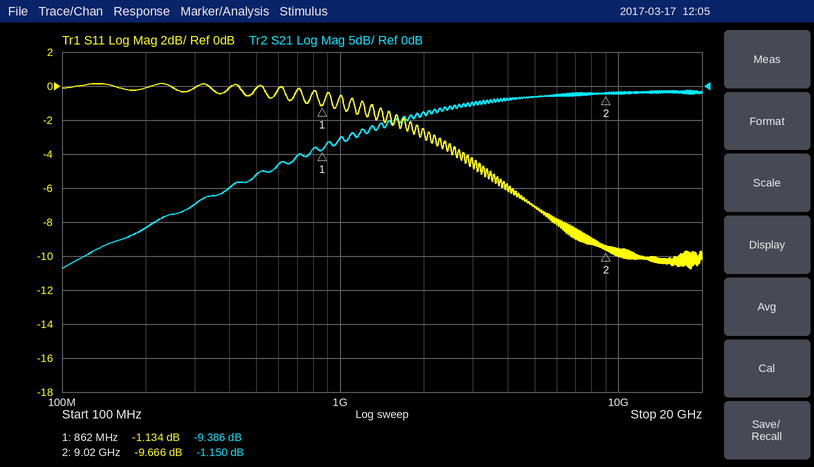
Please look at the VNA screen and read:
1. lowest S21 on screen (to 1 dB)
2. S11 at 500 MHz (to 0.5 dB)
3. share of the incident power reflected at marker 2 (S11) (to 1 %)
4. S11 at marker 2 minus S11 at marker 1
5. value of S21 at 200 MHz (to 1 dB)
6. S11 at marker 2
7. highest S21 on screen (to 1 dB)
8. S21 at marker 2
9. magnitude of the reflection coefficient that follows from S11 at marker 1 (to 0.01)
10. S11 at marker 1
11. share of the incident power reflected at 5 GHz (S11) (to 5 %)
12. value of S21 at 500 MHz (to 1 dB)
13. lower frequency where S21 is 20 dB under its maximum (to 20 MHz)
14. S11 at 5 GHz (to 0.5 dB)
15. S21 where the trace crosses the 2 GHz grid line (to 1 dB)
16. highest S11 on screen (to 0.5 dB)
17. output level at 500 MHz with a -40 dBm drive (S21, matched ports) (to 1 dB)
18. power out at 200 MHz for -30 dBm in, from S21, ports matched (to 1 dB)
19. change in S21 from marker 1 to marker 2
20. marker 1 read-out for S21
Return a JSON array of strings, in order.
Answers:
["-27 dB", "0.0 dB", "11 %", "-8.532 dB", "-21 dB", "-9.666 dB", "-1 dB", "-1.150 dB", "0.88", "-1.134 dB", "20 %", "-13 dB", "200 MHz", "-7.0 dB", "-4 dB", "0.0 dB", "-53 dBm", "-51 dBm", "8.236 dB", "-9.386 dB"]
